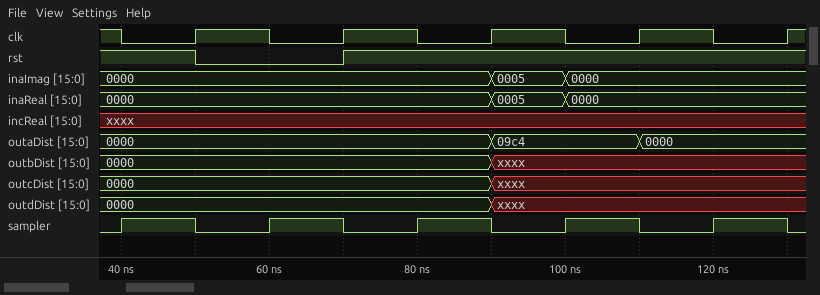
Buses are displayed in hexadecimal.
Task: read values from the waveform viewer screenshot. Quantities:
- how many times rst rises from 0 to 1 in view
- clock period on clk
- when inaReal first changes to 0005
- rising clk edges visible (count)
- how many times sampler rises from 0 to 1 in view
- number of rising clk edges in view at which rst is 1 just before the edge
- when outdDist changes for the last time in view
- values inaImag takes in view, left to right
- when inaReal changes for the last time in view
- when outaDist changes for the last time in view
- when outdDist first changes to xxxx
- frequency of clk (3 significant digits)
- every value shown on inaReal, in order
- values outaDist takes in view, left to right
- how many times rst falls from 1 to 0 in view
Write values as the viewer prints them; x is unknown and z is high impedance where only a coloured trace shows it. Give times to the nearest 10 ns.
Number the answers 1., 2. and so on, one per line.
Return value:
1. 1
2. 20 ns
3. 90 ns
4. 5
5. 5
6. 4
7. 90 ns
8. 0000, 0005, 0000
9. 100 ns
10. 110 ns
11. 90 ns
12. 50.0 MHz
13. 0000, 0005, 0000
14. 0000, 09c4, 0000
15. 1
